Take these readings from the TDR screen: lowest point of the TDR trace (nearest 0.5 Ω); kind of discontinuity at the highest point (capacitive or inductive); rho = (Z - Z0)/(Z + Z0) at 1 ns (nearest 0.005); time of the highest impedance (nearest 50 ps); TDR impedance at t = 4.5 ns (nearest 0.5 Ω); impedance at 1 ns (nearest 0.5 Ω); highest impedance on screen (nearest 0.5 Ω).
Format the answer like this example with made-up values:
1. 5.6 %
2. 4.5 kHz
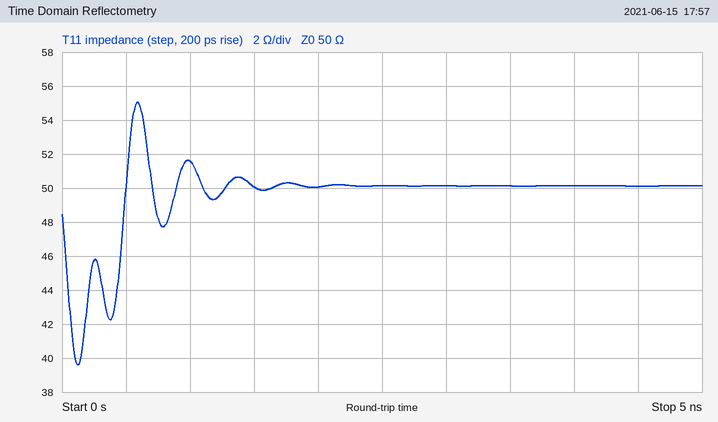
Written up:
1. 39.5 Ω
2. inductive
3. +0.015
4. 600 ps
5. 50.0 Ω
6. 51.5 Ω
7. 55.0 Ω
